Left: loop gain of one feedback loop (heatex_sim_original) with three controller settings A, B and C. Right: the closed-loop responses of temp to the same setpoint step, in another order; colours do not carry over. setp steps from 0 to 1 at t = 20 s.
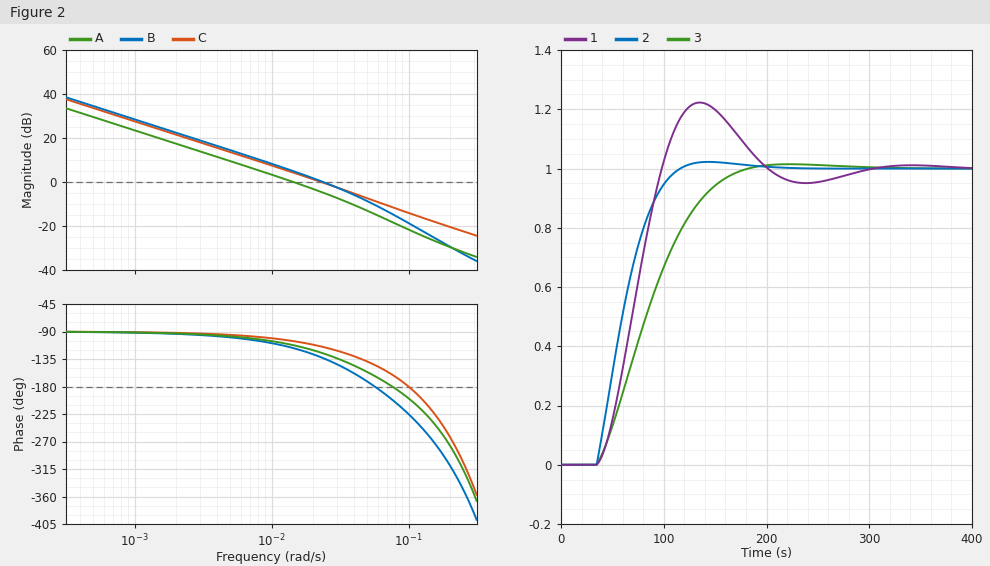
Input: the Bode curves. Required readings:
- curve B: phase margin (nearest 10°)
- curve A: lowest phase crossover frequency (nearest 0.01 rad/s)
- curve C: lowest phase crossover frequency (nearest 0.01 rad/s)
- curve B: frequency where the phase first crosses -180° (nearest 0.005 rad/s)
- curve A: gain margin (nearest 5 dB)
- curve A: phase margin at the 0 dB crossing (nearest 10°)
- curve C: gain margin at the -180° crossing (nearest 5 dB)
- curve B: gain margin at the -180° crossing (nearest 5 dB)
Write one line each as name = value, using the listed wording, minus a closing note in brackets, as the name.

curve B: phase margin = 50°
curve A: lowest phase crossover frequency = 0.08 rad/s
curve C: lowest phase crossover frequency = 0.10 rad/s
curve B: frequency where the phase first crosses -180° = 0.055 rad/s
curve A: gain margin = 20 dB
curve A: phase margin at the 0 dB crossing = 70°
curve C: gain margin at the -180° crossing = 15 dB
curve B: gain margin at the -180° crossing = 10 dB
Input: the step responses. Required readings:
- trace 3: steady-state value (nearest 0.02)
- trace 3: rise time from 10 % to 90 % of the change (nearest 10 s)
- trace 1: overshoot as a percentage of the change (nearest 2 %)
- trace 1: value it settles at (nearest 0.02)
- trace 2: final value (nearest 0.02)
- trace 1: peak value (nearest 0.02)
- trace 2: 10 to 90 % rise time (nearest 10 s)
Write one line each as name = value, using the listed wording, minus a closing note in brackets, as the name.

trace 3: steady-state value = 1.00
trace 3: rise time from 10 % to 90 % of the change = 90 s
trace 1: overshoot as a percentage of the change = 22 %
trace 1: value it settles at = 1.00
trace 2: final value = 1.00
trace 1: peak value = 1.22
trace 2: 10 to 90 % rise time = 50 s
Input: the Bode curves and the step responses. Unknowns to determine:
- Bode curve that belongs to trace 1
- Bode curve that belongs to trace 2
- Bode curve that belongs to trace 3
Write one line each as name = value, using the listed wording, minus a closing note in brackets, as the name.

Bode curve that belongs to trace 1 = B
Bode curve that belongs to trace 2 = C
Bode curve that belongs to trace 3 = A
